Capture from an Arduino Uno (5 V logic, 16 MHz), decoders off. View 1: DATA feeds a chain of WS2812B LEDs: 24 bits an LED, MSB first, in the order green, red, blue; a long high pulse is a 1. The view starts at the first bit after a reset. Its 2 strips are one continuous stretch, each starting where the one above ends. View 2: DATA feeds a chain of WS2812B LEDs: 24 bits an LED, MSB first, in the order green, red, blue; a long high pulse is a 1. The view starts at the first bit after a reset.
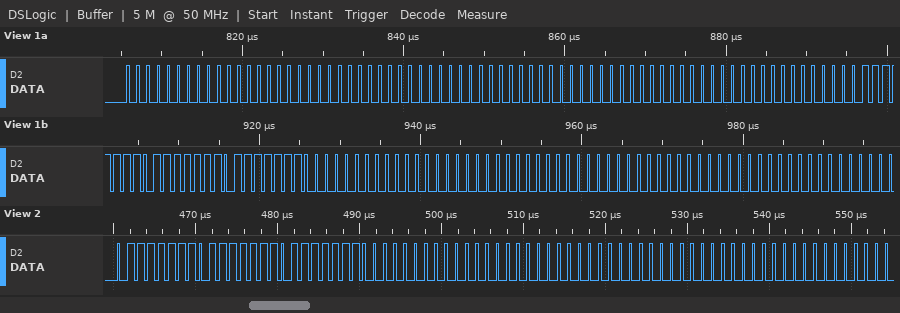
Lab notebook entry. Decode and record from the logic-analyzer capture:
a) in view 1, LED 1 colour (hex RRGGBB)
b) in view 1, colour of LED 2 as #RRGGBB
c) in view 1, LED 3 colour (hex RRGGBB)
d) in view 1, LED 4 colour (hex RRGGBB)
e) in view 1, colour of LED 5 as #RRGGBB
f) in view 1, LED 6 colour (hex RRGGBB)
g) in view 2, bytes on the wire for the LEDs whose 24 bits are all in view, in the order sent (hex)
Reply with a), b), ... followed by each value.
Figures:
a) #000000
b) #000000
c) #000000
d) #7F7F7F
e) #000000
f) #000000
g) 7F 7F 7F 00 00 00 00 00 00
